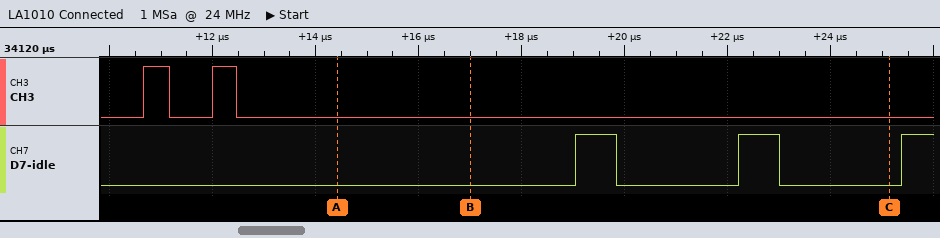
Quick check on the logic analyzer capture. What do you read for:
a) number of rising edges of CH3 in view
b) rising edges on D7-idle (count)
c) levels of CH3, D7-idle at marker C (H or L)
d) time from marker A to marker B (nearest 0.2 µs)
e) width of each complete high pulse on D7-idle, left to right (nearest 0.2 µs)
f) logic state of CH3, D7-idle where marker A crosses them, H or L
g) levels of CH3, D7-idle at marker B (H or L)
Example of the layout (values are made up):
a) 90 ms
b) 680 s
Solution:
a) 2
b) 3
c) CH3=L, D7-idle=L
d) 2.6 µs
e) 0.8 µs, 0.8 µs
f) CH3=L, D7-idle=L
g) CH3=L, D7-idle=L
